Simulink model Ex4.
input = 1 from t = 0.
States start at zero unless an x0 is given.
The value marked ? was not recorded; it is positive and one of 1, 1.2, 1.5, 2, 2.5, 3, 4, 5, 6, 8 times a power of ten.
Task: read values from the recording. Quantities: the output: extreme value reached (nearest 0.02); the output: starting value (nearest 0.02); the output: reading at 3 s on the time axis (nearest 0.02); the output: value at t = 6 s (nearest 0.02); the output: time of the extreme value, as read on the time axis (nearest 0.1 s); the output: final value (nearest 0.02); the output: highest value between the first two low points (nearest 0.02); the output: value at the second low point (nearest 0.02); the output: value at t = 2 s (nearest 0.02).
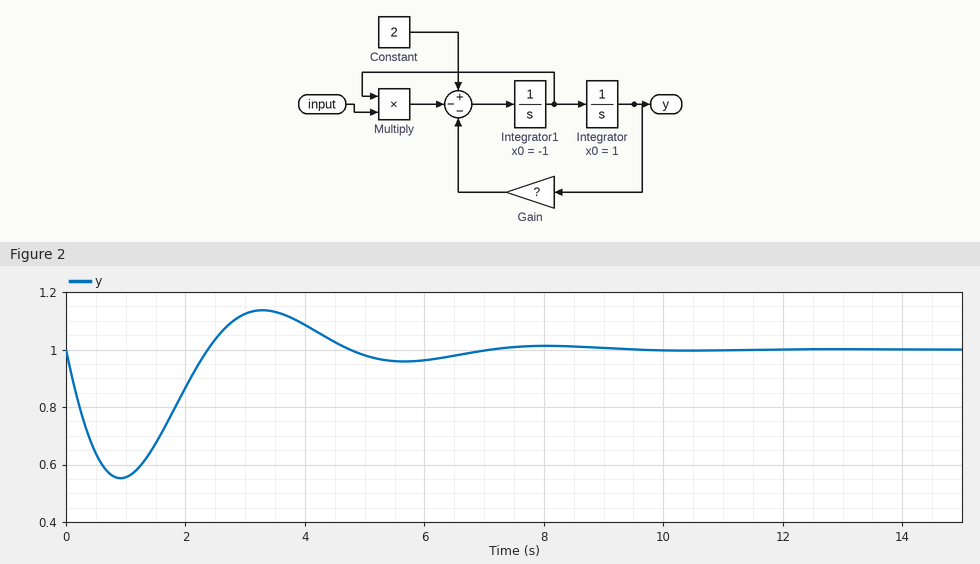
0.56
1.00
1.12
0.96
0.9 s
1.00
1.14
0.96
0.86
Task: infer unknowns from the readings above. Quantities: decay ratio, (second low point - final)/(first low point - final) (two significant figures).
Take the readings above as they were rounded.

0.091
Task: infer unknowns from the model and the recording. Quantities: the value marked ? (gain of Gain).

2
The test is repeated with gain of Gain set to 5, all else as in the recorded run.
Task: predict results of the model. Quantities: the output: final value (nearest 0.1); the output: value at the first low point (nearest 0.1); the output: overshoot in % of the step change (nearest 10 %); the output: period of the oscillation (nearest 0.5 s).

0.4
0.0
60 %
3.0 s
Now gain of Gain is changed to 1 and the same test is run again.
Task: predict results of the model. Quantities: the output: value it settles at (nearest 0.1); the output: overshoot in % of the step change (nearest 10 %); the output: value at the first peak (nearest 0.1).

2.0
20 %
2.2
